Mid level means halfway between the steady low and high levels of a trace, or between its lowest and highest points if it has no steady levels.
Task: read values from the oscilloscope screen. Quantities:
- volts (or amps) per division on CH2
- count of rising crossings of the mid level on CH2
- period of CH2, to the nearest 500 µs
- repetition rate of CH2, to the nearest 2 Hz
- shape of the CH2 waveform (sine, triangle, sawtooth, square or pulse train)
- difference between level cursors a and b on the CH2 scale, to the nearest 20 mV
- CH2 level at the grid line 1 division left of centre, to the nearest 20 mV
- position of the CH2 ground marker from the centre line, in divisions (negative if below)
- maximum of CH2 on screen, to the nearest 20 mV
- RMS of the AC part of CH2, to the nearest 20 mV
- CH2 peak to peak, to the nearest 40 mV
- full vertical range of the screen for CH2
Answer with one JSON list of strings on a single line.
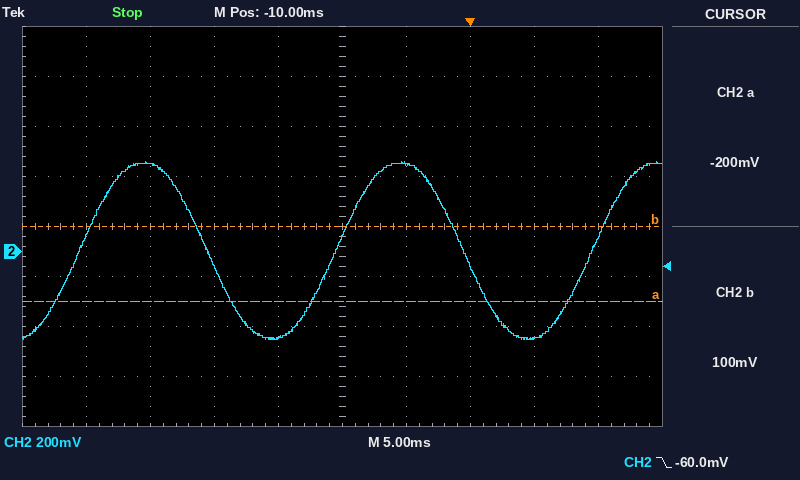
["200 mV", "3", "20.0 ms", "50 Hz", "sine", "300 mV", "-340 mV", "-0.5 div", "360 mV", "260 mV", "720 mV", "1.6 V"]
